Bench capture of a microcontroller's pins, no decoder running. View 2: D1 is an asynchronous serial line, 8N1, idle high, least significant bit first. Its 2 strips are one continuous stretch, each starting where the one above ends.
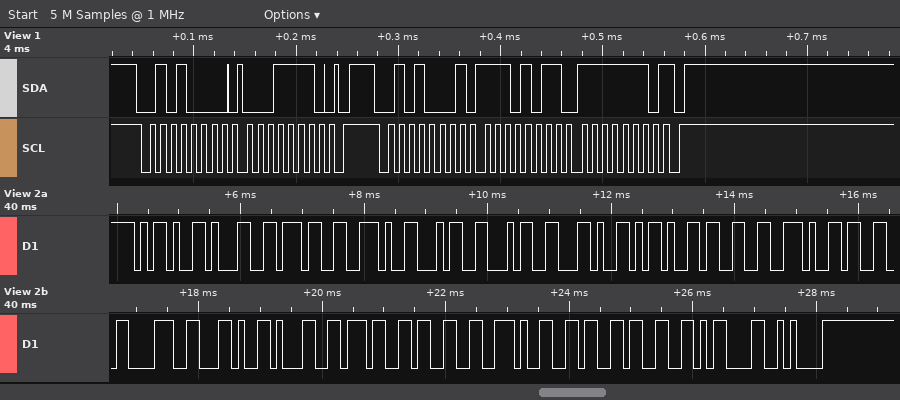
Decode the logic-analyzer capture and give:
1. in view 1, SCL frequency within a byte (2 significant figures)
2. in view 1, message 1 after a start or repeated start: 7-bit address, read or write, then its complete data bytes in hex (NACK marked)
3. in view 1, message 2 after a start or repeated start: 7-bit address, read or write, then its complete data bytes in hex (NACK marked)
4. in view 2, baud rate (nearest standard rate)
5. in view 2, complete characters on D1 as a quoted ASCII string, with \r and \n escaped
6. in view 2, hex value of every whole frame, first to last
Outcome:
100 kHz
0x28 write: 1E
0x28 read: EB FE NACK
9600 baud
"-17.44,-3.38,173.63\r\n"
2D 31 37 2E 34 34 2C 2D 33 2E 33 38 2C 31 37 33 2E 36 33 0D 0A
